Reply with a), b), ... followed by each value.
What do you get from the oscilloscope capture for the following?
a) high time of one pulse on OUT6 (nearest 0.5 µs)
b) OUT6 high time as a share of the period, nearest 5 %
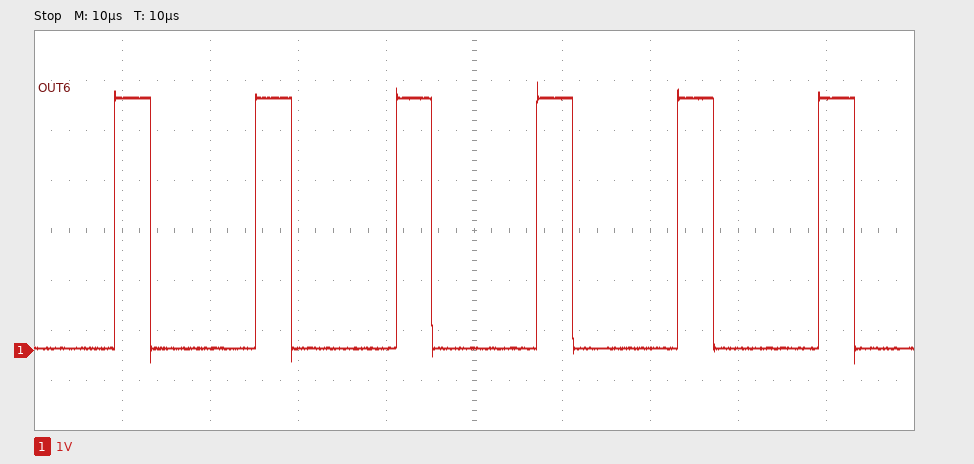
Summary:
a) 4.0 µs
b) 25 %
